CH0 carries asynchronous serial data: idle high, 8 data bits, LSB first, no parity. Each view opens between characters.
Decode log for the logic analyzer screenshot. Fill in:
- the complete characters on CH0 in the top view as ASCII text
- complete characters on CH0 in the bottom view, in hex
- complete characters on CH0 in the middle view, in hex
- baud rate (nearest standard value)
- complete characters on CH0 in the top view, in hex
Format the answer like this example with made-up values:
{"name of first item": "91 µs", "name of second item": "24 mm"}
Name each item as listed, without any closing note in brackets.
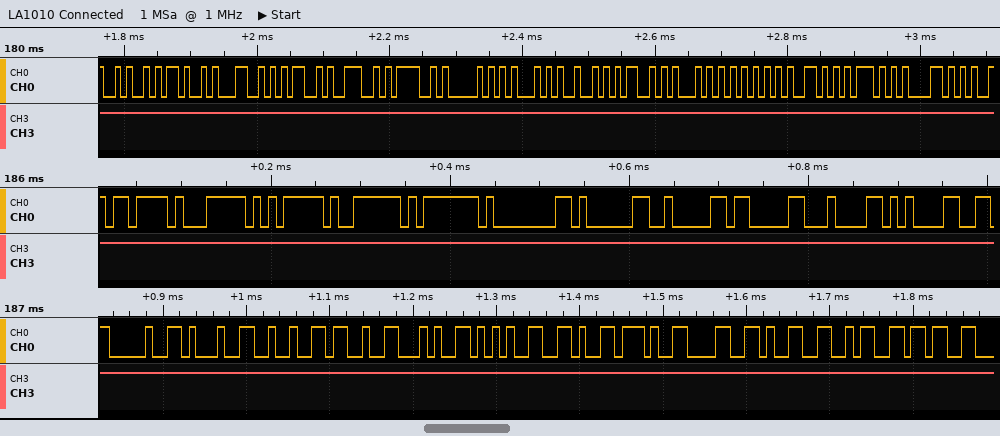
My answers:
{"the complete characters on CH0 in the top view as ASCII text": "\"JKLMNOPQRSTUVWX\"", "complete characters on CH0 in the bottom view, in hex": "90, 91, 92, 93, 94, 95, 96, 97, 98, 99, 9A, 9B", "complete characters on CH0 in the middle view, in hex": "7B, 7C, 7D, 7E, 7F, 80, 81, 82, 83, 84, 85", "baud rate": "115200 baud", "complete characters on CH0 in the top view, in hex": "4A, 4B, 4C, 4D, 4E, 4F, 50, 51, 52, 53, 54, 55, 56, 57, 58"}
